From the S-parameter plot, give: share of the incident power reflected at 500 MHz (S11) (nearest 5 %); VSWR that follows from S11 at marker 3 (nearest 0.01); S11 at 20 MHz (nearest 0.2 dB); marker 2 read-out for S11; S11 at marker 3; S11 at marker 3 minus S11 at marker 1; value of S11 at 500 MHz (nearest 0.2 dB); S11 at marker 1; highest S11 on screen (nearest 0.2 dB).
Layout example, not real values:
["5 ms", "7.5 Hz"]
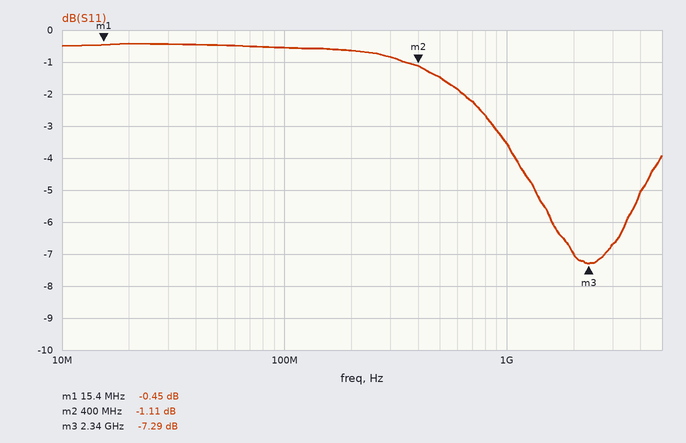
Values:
["70 %", "2.52", "-0.4 dB", "-1.11 dB", "-7.29 dB", "-6.84 dB", "-1.4 dB", "-0.45 dB", "-0.4 dB"]
